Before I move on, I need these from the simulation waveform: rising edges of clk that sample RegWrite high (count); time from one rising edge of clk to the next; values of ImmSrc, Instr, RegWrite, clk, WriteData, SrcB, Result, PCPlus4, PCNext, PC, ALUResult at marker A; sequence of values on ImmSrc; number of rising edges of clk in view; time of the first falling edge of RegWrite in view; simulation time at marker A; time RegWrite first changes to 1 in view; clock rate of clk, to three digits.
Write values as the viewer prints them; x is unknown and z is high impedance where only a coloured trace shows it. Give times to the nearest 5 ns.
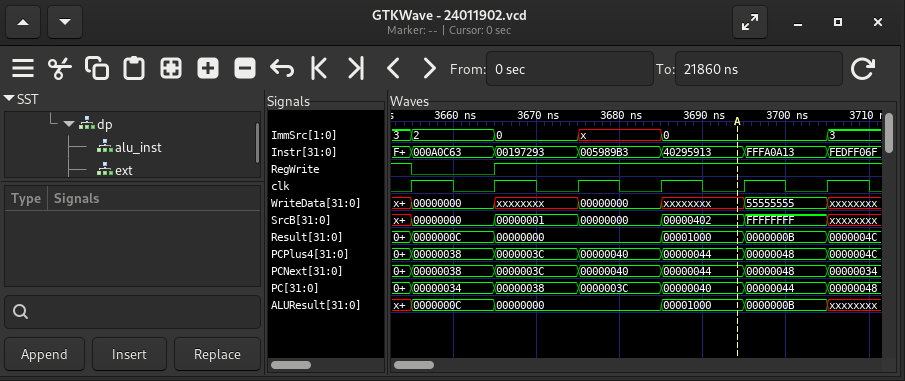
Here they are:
5
10 ns
ImmSrc=0, Instr=40295913, RegWrite=1, clk=0, WriteData=xxxxxxxx, SrcB=00000402, Result=00001000, PCPlus4=00000044, PCNext=00000044, PC=00000040, ALUResult=00001000
3, 2, 0, x, 0, 3
6
3655 ns
3695 ns
3665 ns
100 MHz
